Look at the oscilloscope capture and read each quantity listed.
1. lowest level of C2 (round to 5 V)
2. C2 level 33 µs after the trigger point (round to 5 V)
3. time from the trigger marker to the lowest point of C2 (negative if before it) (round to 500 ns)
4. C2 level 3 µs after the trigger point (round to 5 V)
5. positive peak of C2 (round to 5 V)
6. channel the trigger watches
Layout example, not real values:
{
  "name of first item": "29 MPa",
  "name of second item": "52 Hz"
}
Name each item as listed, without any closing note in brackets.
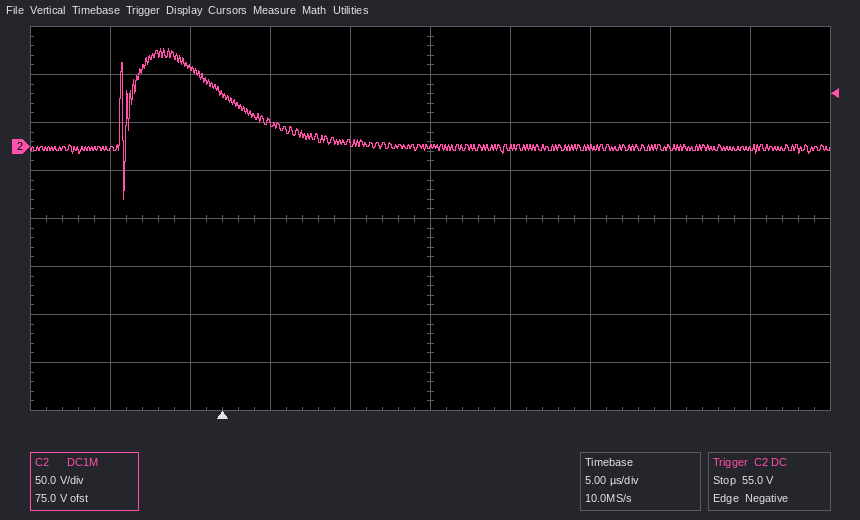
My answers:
{
  "lowest level of C2": "-55 V",
  "C2 level 33 µs after the trigger point": "0 V",
  "time from the trigger marker to the lowest point of C2 (negative if before it)": "-6.0 µs",
  "C2 level 3 µs after the trigger point": "25 V",
  "positive peak of C2": "100 V",
  "channel the trigger watches": "C2"
}
